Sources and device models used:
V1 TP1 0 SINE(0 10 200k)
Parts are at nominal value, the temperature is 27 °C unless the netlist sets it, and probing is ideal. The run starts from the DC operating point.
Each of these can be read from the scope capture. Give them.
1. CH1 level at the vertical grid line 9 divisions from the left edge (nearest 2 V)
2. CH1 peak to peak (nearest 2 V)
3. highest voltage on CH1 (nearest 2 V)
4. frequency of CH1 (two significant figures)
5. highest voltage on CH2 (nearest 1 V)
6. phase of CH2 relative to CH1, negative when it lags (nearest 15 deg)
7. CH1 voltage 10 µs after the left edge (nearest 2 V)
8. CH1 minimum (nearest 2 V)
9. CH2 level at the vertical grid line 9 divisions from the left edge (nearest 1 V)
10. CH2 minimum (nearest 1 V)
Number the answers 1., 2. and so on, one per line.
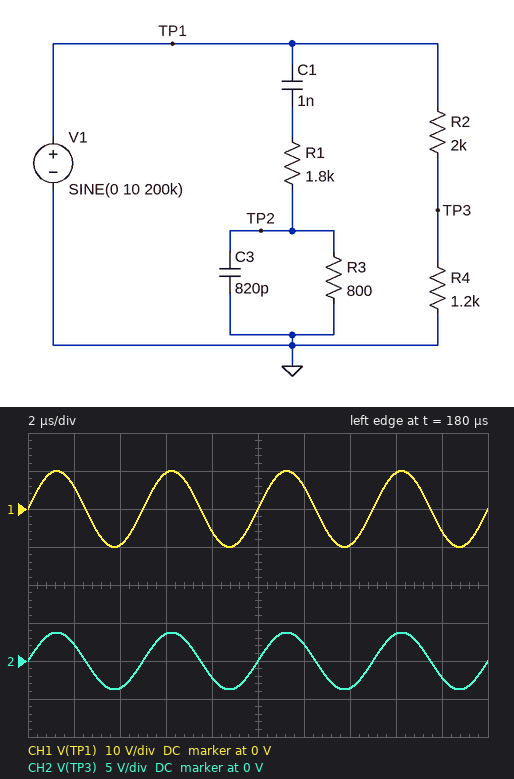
1. -6 V
2. 20 V
3. 10 V
4. 200 kHz
5. 4 V
6. 0 deg
7. 0 V
8. -10 V
9. -2 V
10. -4 V
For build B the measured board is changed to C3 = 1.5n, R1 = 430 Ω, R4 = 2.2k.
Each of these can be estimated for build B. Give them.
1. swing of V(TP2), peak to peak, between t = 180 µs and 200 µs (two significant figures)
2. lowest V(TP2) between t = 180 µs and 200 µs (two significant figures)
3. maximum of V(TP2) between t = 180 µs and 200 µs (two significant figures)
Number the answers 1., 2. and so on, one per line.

1. 6.6 V
2. -3.3 V
3. 3.3 V
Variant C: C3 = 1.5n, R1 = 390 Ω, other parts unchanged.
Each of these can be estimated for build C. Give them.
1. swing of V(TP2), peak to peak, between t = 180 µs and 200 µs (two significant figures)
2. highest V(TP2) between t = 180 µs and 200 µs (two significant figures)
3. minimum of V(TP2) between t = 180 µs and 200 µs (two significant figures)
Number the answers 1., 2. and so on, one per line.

1. 6.7 V
2. 3.3 V
3. -3.3 V
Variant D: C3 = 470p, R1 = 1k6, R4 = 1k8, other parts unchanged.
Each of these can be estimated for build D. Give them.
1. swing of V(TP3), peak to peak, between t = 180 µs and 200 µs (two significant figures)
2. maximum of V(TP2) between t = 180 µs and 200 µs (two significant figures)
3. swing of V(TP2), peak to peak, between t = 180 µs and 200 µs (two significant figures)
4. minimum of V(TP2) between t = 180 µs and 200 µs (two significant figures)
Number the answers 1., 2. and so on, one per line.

1. 9.5 V
2. 2.9 V
3. 5.8 V
4. -2.9 V
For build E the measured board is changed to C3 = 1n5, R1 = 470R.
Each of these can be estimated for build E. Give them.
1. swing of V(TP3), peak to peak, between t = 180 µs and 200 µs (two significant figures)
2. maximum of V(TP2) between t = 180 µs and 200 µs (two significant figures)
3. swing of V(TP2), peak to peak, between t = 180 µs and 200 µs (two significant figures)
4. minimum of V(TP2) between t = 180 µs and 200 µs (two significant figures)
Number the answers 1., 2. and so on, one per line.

1. 7.5 V
2. 3.2 V
3. 6.5 V
4. -3.2 V
